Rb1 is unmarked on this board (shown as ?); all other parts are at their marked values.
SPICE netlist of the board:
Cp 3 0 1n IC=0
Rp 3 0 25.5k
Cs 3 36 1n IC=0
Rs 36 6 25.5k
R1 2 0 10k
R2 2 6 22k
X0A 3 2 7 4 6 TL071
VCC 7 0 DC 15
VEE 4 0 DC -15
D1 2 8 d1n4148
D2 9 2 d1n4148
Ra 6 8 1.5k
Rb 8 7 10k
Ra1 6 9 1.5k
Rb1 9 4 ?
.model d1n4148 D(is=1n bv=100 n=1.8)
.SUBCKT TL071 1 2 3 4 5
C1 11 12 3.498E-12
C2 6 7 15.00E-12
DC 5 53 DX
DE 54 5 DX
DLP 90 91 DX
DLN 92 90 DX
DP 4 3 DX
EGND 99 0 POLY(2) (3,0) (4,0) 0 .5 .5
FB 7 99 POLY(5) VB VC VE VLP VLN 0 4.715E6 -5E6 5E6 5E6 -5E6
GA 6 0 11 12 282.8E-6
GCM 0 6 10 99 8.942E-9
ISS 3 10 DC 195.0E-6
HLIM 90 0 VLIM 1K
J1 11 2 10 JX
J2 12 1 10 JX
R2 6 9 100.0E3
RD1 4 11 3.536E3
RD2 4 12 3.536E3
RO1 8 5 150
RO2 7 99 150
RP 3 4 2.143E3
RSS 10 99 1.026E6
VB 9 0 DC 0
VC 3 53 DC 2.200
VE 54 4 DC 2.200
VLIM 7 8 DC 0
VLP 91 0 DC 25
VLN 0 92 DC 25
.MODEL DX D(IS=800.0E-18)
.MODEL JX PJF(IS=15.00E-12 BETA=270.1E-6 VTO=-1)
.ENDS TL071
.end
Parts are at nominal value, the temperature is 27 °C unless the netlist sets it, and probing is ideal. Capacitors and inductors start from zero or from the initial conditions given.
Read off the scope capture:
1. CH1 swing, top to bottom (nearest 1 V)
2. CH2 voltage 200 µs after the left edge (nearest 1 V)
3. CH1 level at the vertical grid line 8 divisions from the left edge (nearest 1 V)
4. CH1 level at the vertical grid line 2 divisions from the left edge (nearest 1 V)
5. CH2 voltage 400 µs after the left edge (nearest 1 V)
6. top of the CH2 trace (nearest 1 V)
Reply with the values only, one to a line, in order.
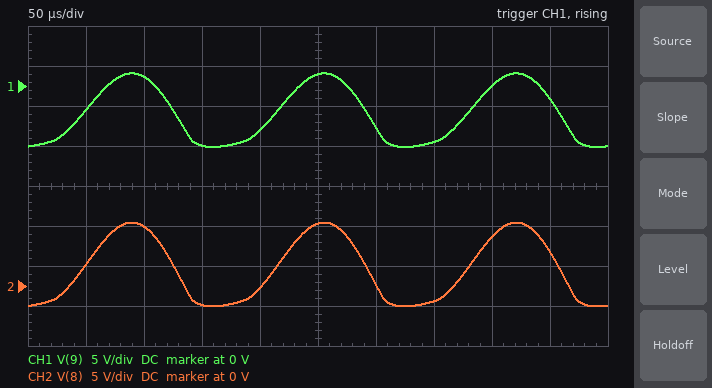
9 V
0 V
0 V
1 V
6 V
8 V
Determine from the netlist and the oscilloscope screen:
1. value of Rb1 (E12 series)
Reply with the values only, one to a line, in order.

4.7 kΩ
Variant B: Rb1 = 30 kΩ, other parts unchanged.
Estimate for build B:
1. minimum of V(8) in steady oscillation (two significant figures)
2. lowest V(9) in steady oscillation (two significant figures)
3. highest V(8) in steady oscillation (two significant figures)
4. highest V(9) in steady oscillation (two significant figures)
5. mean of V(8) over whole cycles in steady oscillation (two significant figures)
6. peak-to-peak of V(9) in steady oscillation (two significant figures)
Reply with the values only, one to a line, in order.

-460 mV
-3.4 V
3.8 V
1.3 V
1.9 V
4.7 V
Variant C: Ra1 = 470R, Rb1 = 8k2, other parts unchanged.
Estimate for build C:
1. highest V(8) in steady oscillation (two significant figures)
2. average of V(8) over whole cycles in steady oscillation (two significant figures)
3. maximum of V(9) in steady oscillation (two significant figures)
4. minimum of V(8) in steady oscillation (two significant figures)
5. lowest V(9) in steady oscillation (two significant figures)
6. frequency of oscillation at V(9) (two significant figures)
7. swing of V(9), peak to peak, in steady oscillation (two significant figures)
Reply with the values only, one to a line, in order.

4.0 V
1.9 V
1.4 V
-680 mV
-3.7 V
6.0 kHz
5.1 V
